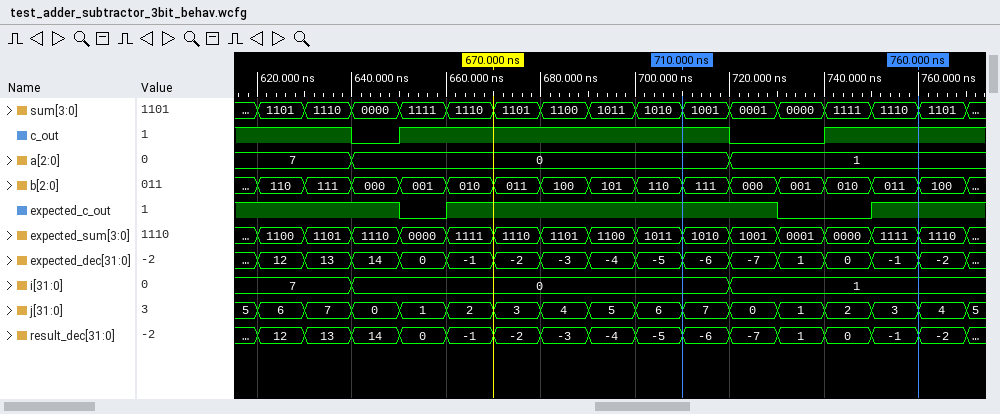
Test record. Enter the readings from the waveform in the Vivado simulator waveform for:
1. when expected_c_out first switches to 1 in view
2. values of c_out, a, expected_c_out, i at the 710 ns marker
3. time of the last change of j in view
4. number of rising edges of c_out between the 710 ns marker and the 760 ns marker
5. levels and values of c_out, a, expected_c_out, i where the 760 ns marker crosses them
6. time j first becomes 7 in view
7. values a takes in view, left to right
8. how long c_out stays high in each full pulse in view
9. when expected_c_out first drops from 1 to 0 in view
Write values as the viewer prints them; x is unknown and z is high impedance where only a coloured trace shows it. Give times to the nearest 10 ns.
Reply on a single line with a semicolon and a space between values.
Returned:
660 ns; c_out=1, a=0, expected_c_out=1, i=0; 770 ns; 1; c_out=1, a=1, expected_c_out=1, i=1; 630 ns; 7, 0, 1; 70 ns; 650 ns
